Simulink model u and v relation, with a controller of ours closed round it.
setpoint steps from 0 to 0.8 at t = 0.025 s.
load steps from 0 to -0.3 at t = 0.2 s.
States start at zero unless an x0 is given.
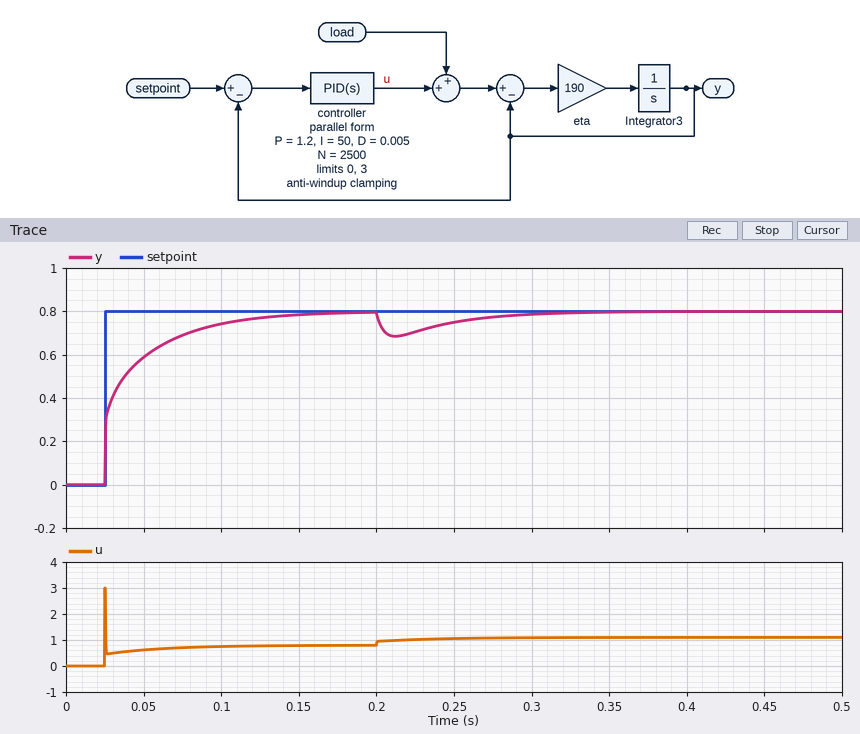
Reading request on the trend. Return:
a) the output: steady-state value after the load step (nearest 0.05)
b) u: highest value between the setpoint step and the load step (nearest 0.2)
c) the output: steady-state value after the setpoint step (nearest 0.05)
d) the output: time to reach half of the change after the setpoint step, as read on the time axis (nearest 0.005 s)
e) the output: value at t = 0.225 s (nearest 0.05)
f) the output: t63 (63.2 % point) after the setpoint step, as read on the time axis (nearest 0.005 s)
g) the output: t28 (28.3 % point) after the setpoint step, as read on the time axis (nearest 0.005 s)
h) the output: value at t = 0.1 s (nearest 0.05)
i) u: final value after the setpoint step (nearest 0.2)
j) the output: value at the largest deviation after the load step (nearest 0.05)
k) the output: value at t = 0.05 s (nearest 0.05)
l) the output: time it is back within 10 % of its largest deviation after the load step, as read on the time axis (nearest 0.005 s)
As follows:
0.80
3.0
0.80
0.030 s
0.70
0.040 s
0.025 s
0.75
0.8
0.70
0.60
0.310 s
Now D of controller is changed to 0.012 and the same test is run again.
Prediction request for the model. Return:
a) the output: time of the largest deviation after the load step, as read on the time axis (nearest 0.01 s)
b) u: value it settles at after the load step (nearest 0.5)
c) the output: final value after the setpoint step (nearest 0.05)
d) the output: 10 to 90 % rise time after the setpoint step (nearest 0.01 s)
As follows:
0.22 s
1.0
0.80
0.06 s
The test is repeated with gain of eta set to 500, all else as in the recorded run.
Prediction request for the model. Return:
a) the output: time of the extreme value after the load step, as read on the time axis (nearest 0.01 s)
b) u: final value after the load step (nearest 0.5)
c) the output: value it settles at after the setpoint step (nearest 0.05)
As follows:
0.21 s
1.0
0.80
